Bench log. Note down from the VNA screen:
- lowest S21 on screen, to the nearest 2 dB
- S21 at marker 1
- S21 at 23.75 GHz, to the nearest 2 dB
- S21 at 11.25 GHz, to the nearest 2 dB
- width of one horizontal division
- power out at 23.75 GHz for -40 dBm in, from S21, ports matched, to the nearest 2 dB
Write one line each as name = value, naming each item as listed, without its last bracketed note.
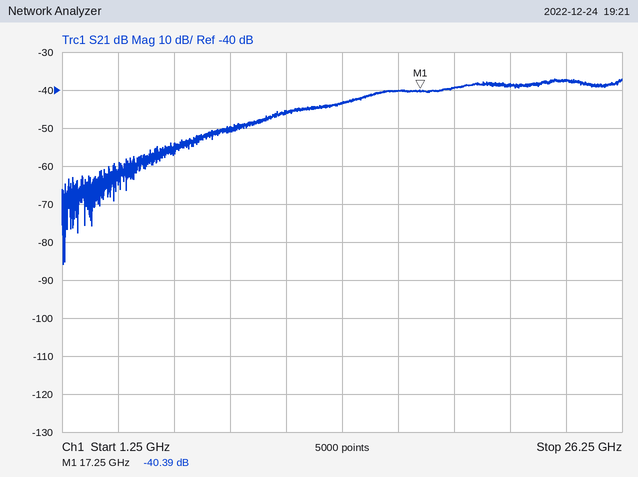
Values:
lowest S21 on screen, to the nearest 2 dB = -86 dB
S21 at marker 1 = -40.39 dB
S21 at 23.75 GHz, to the nearest 2 dB = -38 dB
S21 at 11.25 GHz, to the nearest 2 dB = -46 dB
width of one horizontal division = 2.5 GHz
power out at 23.75 GHz for -40 dBm in, from S21, ports matched, to the nearest 2 dB = -78 dBm
